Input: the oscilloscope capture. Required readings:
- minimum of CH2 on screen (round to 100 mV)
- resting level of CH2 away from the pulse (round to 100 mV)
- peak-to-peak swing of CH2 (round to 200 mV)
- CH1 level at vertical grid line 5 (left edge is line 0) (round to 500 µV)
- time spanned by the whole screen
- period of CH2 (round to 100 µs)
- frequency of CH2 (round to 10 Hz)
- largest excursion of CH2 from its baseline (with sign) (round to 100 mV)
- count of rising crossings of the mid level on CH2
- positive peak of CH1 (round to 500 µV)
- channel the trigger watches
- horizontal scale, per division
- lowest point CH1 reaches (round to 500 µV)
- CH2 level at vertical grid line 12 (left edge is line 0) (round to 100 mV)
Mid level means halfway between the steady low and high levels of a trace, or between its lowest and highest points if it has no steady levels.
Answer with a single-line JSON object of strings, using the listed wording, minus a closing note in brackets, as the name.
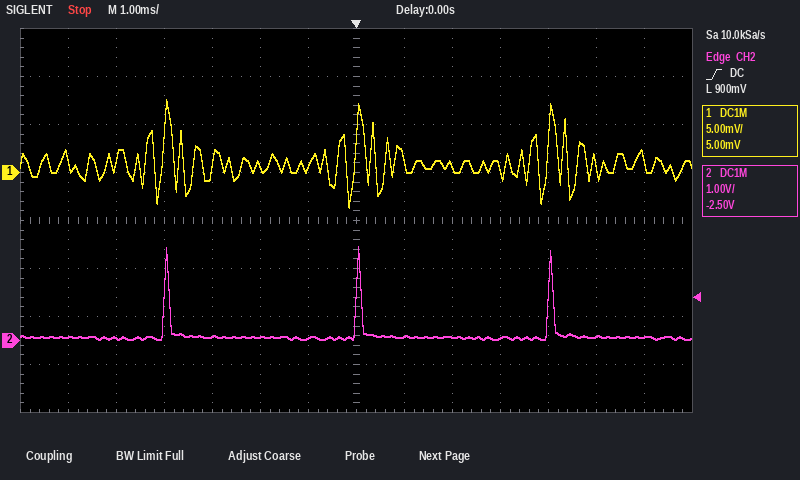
{"minimum of CH2 on screen": "0.0 V", "resting level of CH2 away from the pulse": "100 mV", "peak-to-peak swing of CH2": "2.0 V", "CH1 level at vertical grid line 5 (left edge is line 0)": "500 µV", "time spanned by the whole screen": "14 ms", "period of CH2": "4.0 ms", "frequency of CH2": "250 Hz", "largest excursion of CH2 from its baseline (with sign)": "+1.9 V", "count of rising crossings of the mid level on CH2": "3", "positive peak of CH1": "7.5 mV", "channel the trigger watches": "CH2", "horizontal scale, per division": "1 ms", "lowest point CH1 reaches": "-3.5 mV", "CH2 level at vertical grid line 12 (left edge is line 0)": "100 mV"}
